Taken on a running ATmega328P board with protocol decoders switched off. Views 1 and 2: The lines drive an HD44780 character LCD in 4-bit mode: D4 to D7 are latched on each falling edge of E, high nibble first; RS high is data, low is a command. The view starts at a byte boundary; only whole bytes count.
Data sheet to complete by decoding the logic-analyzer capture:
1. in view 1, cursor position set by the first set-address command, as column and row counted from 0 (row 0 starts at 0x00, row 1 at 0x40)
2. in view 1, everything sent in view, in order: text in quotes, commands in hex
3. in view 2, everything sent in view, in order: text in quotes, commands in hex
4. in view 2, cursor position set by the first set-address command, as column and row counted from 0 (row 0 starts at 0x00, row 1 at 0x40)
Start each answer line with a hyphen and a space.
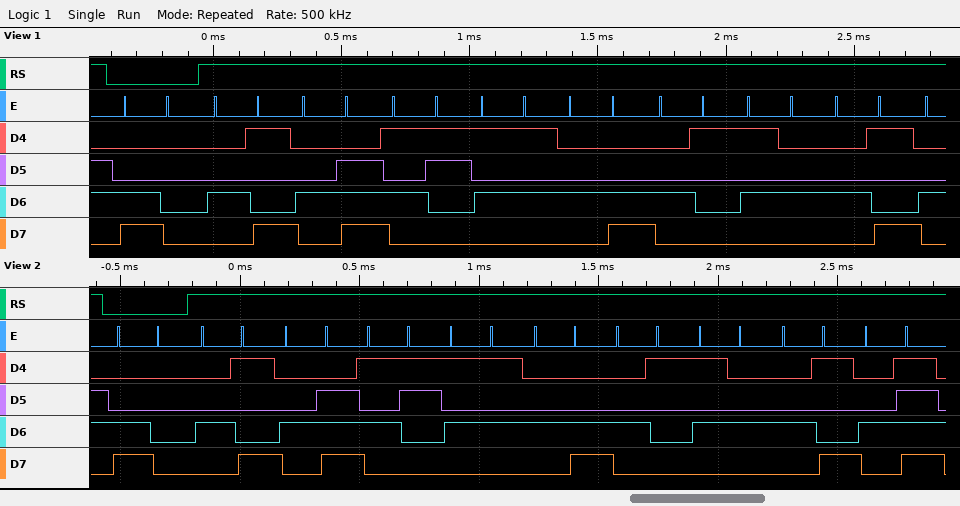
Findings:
- column 0, row 1
- 0xC0 "INSULATI"
- 0xC0 "INSULATIO"
- column 0, row 1
